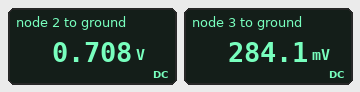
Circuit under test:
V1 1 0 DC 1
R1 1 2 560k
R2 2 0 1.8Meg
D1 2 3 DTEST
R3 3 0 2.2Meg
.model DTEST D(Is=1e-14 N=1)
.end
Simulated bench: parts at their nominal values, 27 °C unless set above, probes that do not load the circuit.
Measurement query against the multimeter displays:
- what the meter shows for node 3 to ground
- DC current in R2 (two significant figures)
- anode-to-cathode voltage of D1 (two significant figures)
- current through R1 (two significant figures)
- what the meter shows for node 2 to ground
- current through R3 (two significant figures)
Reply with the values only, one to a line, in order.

284.1 mV
390 nA
420 mV
520 nA
0.708 V
130 nA
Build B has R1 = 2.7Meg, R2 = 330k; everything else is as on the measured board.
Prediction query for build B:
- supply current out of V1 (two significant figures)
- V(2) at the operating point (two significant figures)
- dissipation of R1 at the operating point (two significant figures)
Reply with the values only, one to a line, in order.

330 nA
110 mV
290 nW
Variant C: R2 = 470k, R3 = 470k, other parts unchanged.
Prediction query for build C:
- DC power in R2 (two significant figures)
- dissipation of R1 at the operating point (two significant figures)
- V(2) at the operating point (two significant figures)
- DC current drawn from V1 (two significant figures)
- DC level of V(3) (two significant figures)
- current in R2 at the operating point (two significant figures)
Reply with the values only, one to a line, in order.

410 nW
560 nW
440 mV
1.0 µA
32 mV
930 nA
